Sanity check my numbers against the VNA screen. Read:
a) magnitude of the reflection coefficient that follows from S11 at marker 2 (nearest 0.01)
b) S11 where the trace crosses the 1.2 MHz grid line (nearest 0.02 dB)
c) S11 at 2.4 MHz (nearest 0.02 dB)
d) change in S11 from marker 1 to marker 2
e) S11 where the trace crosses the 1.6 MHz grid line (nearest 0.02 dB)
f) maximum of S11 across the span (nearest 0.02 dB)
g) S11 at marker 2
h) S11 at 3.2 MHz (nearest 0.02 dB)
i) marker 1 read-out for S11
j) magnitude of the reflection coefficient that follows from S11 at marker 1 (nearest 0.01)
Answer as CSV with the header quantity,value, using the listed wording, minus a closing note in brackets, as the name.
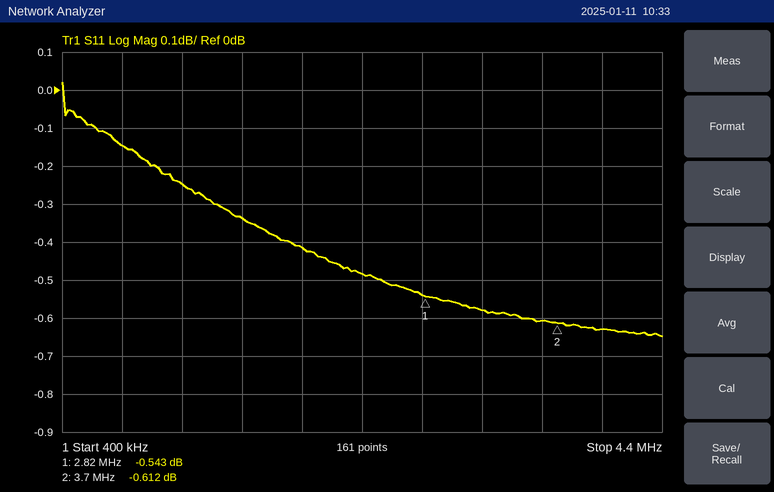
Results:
quantity,value
magnitude of the reflection coefficient that follows from S11 at marker 2,0.93
S11 where the trace crosses the 1.2 MHz grid line,-0.24 dB
S11 at 2.4 MHz,-0.48 dB
change in S11 from marker 1 to marker 2,-0.069 dB
S11 where the trace crosses the 1.6 MHz grid line,-0.34 dB
maximum of S11 across the span,0.02 dB
S11 at marker 2,-0.612 dB
S11 at 3.2 MHz,-0.58 dB
marker 1 read-out for S11,-0.543 dB
magnitude of the reflection coefficient that follows from S11 at marker 1,0.94
